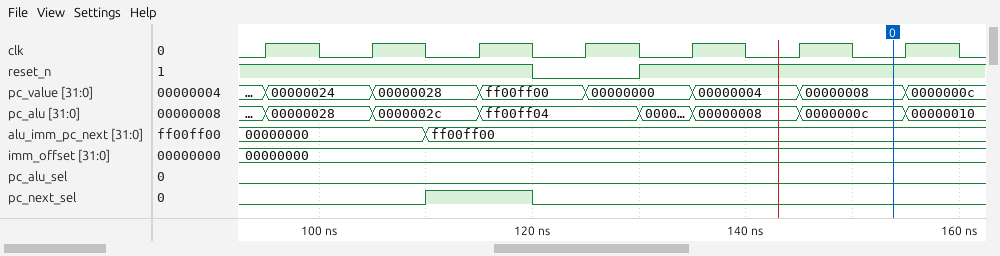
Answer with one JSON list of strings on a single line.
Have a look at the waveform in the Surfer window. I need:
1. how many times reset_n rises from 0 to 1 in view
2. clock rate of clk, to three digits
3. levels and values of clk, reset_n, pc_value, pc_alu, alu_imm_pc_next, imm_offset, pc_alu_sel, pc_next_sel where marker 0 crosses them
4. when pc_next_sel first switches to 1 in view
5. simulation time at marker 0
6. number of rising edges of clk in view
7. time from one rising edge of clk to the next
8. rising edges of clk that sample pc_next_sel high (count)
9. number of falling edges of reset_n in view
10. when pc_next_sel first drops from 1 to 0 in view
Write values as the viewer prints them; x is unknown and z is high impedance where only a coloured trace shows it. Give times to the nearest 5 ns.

["1", "100 MHz", "clk=0, reset_n=1, pc_value=00000008, pc_alu=0000000c, alu_imm_pc_next=ff00ff00, imm_offset=00000000, pc_alu_sel=0, pc_next_sel=0", "110 ns", "155 ns", "7", "10 ns", "1", "1", "120 ns"]
